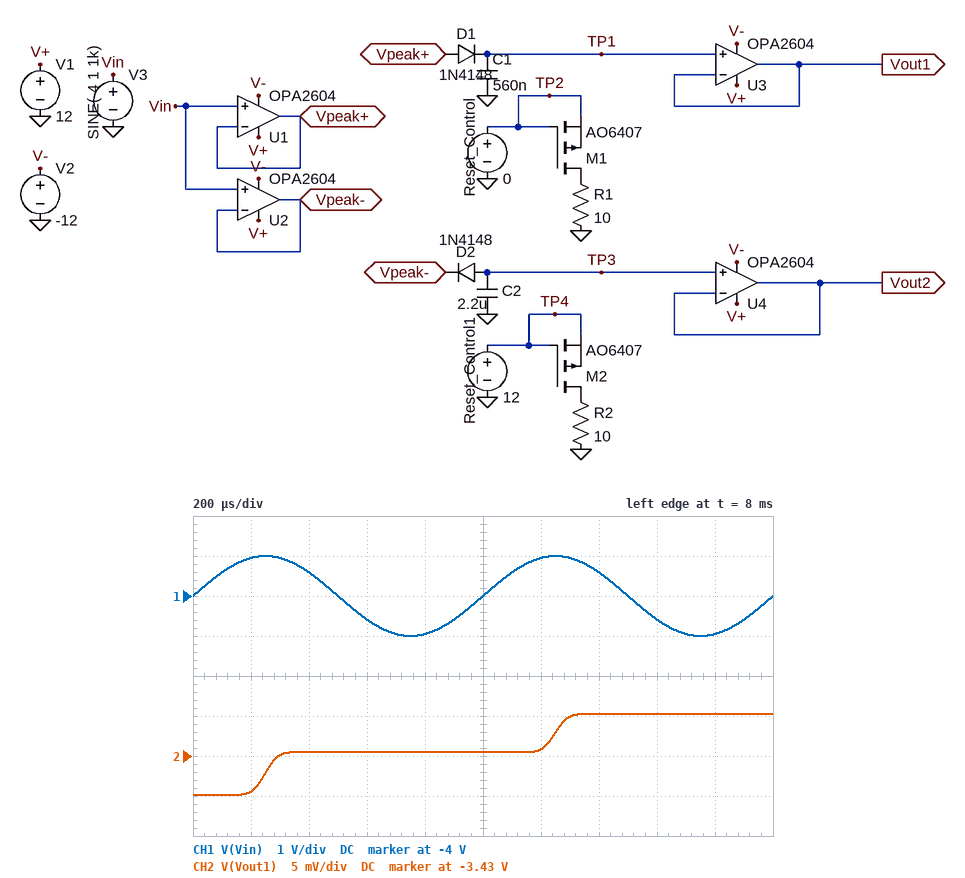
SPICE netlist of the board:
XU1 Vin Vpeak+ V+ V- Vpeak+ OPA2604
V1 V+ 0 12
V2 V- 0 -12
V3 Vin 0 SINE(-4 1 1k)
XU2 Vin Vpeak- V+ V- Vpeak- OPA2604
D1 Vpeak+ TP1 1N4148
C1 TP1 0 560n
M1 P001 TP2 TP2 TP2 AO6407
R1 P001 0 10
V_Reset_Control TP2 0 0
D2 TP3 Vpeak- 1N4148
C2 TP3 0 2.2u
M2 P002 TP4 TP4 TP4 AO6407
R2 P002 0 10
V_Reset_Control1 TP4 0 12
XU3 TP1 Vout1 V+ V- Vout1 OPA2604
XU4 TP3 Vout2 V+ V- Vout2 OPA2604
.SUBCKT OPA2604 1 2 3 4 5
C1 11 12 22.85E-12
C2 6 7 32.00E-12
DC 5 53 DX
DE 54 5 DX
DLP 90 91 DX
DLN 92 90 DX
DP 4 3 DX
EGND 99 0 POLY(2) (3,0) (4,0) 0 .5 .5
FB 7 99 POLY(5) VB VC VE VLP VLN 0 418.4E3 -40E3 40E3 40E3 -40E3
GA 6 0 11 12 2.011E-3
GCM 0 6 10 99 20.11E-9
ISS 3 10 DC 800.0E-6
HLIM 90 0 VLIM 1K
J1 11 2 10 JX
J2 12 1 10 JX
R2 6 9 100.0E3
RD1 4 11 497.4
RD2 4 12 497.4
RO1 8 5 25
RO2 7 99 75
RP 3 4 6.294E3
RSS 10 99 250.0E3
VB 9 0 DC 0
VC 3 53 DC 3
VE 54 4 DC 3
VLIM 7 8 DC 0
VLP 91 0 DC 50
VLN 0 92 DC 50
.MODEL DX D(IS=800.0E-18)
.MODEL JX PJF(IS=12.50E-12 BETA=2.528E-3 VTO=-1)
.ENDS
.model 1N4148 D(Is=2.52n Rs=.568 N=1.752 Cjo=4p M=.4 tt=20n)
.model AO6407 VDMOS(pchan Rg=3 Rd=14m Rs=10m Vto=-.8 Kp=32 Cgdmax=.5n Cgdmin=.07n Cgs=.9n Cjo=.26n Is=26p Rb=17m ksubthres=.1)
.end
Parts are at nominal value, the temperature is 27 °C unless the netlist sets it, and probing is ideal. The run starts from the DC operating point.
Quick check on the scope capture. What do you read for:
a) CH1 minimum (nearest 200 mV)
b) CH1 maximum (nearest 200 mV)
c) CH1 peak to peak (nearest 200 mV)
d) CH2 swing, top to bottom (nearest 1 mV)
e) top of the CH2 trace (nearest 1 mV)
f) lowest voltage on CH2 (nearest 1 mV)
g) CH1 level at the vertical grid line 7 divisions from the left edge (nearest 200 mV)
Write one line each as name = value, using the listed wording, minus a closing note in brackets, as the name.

CH1 minimum = -5.0 V
CH1 maximum = -3.0 V
CH1 peak to peak = 2.0 V
CH2 swing, top to bottom = 10 mV
top of the CH2 trace = -3.425 V
lowest voltage on CH2 = -3.435 V
CH1 level at the vertical grid line 7 divisions from the left edge = -3.4 V
